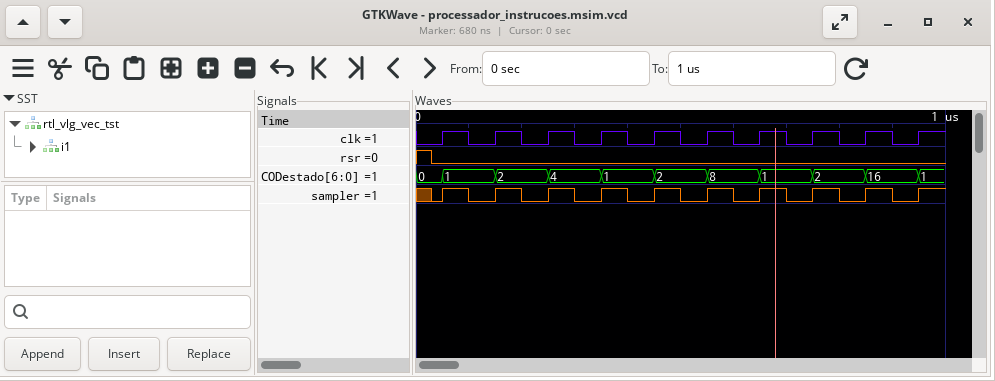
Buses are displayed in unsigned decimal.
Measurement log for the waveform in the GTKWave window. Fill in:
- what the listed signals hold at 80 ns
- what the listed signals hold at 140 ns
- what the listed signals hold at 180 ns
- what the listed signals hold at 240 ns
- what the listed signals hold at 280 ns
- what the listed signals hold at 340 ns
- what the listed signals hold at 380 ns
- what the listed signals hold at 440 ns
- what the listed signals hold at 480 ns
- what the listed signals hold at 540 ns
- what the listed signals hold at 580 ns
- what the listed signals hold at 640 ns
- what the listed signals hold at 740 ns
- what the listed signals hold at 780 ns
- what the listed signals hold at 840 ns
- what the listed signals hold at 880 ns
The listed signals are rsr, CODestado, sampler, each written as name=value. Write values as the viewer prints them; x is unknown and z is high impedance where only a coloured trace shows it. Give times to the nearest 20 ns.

rsr=0, CODestado=1, sampler=1
rsr=0, CODestado=1, sampler=0
rsr=0, CODestado=2, sampler=1
rsr=0, CODestado=2, sampler=0
rsr=0, CODestado=4, sampler=1
rsr=0, CODestado=4, sampler=0
rsr=0, CODestado=1, sampler=1
rsr=0, CODestado=1, sampler=0
rsr=0, CODestado=2, sampler=1
rsr=0, CODestado=2, sampler=0
rsr=0, CODestado=8, sampler=1
rsr=0, CODestado=8, sampler=0
rsr=0, CODestado=1, sampler=0
rsr=0, CODestado=2, sampler=1
rsr=0, CODestado=2, sampler=0
rsr=0, CODestado=16, sampler=1
